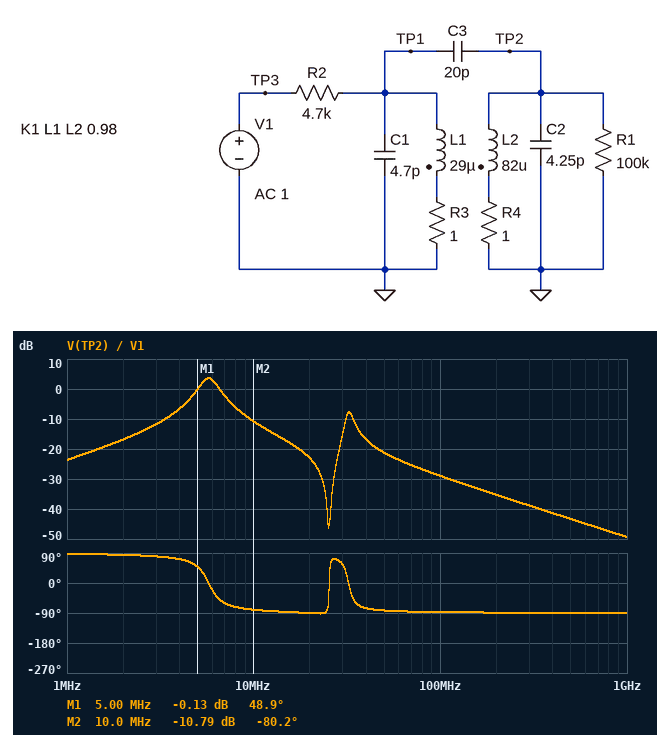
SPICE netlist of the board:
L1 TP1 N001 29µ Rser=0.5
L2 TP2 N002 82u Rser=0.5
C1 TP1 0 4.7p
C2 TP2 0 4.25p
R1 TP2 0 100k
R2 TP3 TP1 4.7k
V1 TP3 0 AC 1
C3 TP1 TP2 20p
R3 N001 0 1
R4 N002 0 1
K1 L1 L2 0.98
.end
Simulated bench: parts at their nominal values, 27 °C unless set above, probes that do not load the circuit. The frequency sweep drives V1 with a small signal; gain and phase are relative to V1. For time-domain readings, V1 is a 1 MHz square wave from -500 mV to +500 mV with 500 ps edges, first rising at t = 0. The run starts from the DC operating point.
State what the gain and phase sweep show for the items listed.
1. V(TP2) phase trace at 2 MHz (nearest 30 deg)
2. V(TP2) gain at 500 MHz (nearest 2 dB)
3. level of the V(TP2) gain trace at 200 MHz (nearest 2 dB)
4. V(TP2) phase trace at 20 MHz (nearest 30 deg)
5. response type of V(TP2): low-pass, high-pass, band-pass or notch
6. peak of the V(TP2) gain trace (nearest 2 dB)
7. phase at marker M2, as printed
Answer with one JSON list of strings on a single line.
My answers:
["90 deg", "-44 dB", "-36 dB", "-90 deg", "band-pass", "4 dB", "-80.2 deg"]
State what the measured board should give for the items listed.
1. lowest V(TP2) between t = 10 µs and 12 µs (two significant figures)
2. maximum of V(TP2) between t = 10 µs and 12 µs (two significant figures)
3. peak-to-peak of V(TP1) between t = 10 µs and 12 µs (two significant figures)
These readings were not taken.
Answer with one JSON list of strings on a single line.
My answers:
["-310 mV", "310 mV", "450 mV"]
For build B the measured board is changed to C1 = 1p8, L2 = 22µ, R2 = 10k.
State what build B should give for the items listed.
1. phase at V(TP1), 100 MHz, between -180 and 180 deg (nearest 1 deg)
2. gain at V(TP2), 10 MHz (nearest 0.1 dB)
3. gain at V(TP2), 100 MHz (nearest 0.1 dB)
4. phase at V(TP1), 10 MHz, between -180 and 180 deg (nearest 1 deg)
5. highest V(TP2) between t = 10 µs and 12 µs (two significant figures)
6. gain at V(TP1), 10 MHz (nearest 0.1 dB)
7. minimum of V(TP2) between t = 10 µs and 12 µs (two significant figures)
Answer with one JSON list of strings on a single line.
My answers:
["-88 deg", "-8.9 dB", "-32.0 dB", "63 deg", "170 mV", "-7.6 dB", "-170 mV"]
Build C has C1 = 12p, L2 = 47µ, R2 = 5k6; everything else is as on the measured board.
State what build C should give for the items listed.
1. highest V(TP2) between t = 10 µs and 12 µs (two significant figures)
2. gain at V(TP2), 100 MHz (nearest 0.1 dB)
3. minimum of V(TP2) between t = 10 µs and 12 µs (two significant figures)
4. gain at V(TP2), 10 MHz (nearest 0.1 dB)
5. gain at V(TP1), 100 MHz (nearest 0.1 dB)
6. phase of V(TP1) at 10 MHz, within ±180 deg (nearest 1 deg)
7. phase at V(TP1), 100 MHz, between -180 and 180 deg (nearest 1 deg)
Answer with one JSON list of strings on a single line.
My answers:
["230 mV", "-36.5 dB", "-230 mV", "-10.3 dB", "-34.5 dB", "-75 deg", "-89 deg"]
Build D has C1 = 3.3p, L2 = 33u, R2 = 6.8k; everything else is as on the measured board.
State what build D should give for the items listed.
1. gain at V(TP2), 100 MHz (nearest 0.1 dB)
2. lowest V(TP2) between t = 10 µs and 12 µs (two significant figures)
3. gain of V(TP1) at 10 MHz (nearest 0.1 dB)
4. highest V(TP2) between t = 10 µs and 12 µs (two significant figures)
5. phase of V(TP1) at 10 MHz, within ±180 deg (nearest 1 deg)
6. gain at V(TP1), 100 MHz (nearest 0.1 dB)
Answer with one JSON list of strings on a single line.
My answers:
["-30.9 dB", "-240 mV", "-0.9 dB", "240 mV", "13 deg", "-29.0 dB"]
